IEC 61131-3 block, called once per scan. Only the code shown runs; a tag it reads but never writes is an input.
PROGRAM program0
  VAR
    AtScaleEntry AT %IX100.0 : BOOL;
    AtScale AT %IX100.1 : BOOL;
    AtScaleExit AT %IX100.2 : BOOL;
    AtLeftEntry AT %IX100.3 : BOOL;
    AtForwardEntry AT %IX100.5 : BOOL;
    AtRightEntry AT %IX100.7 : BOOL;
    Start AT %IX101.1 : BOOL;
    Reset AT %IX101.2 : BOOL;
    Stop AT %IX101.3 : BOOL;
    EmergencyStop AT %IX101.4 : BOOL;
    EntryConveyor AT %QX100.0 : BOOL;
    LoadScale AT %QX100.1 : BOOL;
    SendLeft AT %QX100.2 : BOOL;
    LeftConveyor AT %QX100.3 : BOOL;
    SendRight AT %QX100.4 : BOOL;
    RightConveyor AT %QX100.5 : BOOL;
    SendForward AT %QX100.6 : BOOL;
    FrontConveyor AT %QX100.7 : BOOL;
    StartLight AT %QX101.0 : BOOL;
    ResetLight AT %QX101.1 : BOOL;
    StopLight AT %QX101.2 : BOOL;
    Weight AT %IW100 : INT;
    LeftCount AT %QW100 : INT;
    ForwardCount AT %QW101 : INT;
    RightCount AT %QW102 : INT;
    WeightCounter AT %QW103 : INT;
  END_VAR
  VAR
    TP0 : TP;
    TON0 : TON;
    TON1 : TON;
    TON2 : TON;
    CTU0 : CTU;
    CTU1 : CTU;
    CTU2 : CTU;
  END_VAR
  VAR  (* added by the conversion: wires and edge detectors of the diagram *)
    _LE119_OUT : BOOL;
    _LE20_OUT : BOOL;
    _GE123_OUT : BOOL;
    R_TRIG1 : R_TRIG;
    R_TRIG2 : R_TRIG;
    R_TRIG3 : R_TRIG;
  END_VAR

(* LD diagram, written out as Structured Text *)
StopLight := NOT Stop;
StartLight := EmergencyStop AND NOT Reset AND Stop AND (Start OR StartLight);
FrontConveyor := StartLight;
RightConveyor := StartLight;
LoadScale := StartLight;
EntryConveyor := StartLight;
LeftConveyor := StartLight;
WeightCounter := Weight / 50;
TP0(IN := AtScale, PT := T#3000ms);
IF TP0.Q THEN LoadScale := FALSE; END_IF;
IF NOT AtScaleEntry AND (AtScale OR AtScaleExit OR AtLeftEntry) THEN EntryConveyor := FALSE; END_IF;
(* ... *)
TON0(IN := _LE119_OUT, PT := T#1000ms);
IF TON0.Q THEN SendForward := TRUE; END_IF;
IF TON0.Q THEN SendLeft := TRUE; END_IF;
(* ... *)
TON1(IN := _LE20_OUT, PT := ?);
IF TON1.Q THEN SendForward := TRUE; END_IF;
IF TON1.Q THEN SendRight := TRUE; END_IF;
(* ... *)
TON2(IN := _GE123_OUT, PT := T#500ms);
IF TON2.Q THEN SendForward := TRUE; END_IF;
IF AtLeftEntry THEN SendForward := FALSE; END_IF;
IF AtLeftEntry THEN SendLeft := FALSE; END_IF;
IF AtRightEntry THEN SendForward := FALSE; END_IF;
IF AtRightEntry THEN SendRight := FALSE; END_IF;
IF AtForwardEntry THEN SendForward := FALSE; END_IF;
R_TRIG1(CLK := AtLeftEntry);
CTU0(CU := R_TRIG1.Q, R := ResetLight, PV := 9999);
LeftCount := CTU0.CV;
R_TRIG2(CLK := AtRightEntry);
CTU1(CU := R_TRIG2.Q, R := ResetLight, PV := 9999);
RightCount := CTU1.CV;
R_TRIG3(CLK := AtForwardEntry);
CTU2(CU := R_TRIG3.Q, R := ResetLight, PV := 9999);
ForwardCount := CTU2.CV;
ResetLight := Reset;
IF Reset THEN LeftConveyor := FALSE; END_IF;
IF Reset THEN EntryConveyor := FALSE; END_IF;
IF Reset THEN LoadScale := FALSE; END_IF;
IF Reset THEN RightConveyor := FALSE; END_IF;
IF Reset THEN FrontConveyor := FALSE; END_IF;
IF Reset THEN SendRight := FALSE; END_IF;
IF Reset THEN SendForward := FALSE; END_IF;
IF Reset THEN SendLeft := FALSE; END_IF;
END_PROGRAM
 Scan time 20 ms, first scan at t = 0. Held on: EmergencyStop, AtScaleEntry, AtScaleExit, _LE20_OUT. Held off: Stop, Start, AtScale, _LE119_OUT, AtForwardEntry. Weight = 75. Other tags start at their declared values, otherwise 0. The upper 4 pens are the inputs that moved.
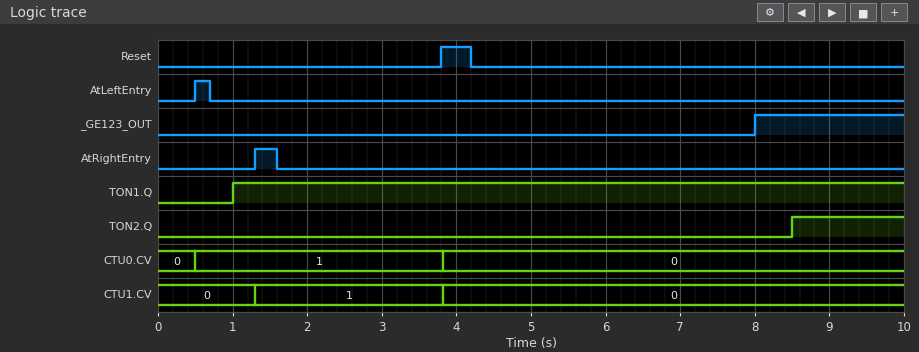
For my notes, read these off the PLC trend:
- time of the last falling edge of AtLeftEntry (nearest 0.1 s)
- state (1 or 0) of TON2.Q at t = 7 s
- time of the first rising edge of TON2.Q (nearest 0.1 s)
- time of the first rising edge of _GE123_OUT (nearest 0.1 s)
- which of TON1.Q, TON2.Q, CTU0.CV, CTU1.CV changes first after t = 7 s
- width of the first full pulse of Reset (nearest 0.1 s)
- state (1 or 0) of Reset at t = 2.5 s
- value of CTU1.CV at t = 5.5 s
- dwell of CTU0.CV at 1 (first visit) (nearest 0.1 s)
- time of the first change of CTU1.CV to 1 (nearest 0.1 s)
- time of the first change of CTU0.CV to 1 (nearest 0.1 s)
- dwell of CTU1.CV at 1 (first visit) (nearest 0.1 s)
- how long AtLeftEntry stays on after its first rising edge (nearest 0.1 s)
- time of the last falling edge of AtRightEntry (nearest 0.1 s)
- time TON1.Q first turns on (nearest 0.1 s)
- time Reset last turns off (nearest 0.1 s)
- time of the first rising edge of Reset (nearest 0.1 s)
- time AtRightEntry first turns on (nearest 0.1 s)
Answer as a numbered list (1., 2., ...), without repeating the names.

1. 0.7 s
2. 0
3. 8.5 s
4. 8.0 s
5. TON2.Q
6. 0.4 s
7. 0
8. 0
9. 3.3 s
10. 1.3 s
11. 0.5 s
12. 2.5 s
13. 0.2 s
14. 1.6 s
15. 1.0 s
16. 4.2 s
17. 3.8 s
18. 1.3 s
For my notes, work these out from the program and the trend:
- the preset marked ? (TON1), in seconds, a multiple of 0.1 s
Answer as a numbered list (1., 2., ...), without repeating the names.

1. 1.0 s
